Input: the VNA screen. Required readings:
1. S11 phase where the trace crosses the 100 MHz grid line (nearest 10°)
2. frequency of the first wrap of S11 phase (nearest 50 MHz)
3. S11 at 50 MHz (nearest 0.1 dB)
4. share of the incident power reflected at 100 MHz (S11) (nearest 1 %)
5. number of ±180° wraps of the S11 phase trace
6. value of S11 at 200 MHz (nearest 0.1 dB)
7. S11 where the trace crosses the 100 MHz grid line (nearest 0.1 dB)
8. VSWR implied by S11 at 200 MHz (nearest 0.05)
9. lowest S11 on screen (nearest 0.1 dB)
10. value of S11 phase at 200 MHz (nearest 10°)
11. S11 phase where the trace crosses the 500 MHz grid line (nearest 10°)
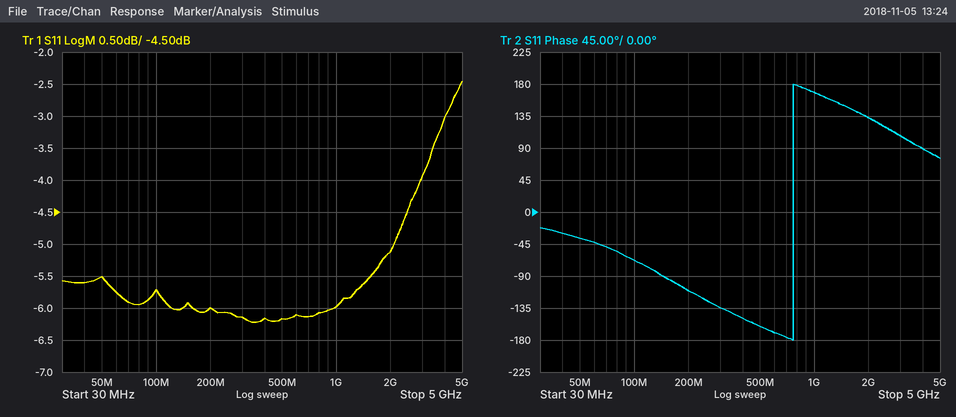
-70°
750 MHz
-5.5 dB
27 %
1
-6.0 dB
-5.7 dB
3.00
-6.2 dB
-110°
-160°
